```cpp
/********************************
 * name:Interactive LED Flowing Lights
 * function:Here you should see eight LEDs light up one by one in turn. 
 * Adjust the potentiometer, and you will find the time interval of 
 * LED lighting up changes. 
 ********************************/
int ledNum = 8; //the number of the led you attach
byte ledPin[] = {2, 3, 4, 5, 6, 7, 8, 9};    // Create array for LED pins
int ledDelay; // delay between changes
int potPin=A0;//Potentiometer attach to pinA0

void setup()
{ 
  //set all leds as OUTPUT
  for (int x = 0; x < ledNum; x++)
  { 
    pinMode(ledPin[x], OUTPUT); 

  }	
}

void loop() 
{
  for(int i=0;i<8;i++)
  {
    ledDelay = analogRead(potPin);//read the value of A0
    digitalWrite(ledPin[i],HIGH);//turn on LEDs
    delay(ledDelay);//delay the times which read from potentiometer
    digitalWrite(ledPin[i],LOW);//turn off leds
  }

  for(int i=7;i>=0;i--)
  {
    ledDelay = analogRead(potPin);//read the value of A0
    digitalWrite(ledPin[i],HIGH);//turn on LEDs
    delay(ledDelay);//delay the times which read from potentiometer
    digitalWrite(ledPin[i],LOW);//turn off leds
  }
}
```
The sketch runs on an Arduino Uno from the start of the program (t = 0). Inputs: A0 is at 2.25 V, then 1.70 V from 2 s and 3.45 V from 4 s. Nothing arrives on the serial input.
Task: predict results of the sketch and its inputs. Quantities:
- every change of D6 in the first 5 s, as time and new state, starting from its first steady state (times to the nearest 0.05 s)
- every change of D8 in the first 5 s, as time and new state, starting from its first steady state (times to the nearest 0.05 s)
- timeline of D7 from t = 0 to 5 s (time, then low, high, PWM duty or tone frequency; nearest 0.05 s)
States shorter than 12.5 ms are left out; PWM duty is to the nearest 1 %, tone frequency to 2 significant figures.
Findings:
0 s low; 1.85 s high; 2.3 s low; 4.75 s high
0 s low; 2.65 s high; 3 s low; 3.7 s high; 4.05 s low
0 s low; 2.3 s high; 2.65 s low; 4.05 s high; 4.75 s low
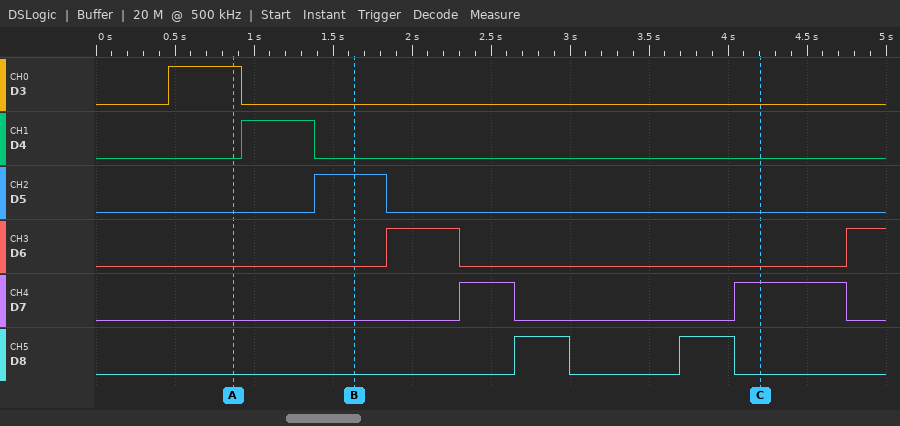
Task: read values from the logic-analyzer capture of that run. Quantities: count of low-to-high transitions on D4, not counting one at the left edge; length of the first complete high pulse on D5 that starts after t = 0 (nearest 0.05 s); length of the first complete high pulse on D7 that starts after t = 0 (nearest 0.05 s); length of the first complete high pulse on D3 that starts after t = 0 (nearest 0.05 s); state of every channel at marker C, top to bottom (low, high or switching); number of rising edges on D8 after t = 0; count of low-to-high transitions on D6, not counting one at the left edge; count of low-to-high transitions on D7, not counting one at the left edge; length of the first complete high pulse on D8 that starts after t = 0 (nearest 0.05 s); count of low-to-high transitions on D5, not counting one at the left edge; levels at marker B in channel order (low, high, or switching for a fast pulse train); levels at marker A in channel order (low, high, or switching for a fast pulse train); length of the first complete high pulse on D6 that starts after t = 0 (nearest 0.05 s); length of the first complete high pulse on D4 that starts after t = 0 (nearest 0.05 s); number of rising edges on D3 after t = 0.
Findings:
1
0.45 s
0.35 s
0.45 s
D3 low, D4 low, D5 low, D6 low, D7 high, D8 low
2
2
2
0.35 s
1
D3 low, D4 low, D5 high, D6 low, D7 low, D8 low
D3 high, D4 low, D5 low, D6 low, D7 low, D8 low
0.45 s
0.45 s
1
